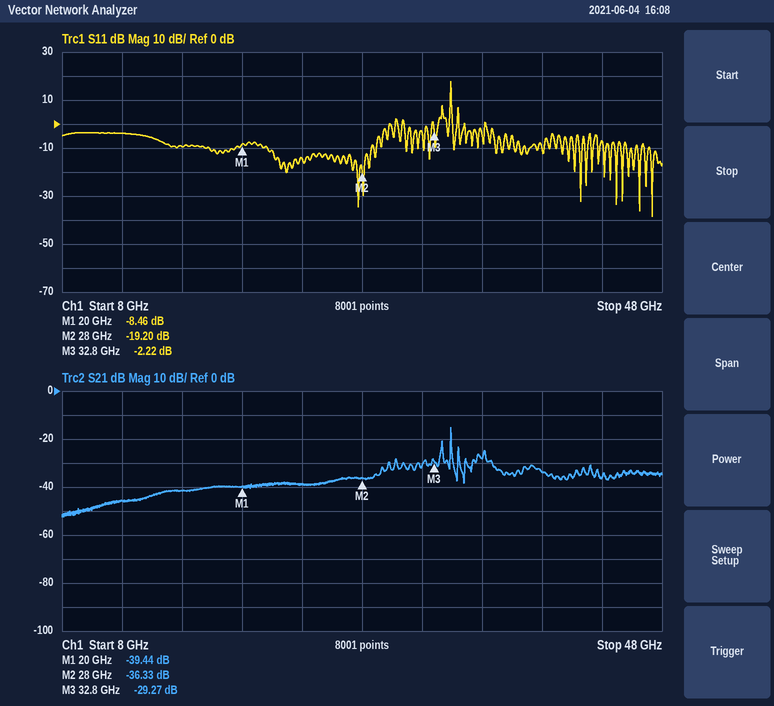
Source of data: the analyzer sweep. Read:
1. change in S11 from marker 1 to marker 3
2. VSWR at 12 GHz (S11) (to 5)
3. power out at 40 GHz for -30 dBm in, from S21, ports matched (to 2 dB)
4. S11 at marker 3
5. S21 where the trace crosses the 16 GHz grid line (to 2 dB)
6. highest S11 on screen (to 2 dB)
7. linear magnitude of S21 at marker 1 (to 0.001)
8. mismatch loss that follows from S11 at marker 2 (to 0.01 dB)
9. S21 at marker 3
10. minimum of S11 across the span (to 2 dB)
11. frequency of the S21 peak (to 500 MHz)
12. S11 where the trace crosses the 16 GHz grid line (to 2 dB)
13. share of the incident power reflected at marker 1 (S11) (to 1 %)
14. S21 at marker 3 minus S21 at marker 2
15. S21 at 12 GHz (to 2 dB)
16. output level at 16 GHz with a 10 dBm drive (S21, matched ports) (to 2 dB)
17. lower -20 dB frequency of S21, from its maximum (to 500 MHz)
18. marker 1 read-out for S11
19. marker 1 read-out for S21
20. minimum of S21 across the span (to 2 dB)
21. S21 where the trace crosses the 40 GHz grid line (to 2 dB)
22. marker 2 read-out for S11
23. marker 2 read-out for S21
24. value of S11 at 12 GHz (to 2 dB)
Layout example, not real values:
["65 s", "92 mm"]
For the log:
["6.24 dB", "5", "-64 dBm", "-2.22 dB", "-42 dB", "18 dB", "0.011", "0.05 dB", "-29.27 dB", "-38 dB", "34.0 GHz", "-10 dB", "14 %", "7.06 dB", "-46 dB", "-32 dBm", "29.0 GHz", "-8.46 dB", "-39.44 dB", "-52 dB", "-34 dB", "-19.20 dB", "-36.33 dB", "-4 dB"]
